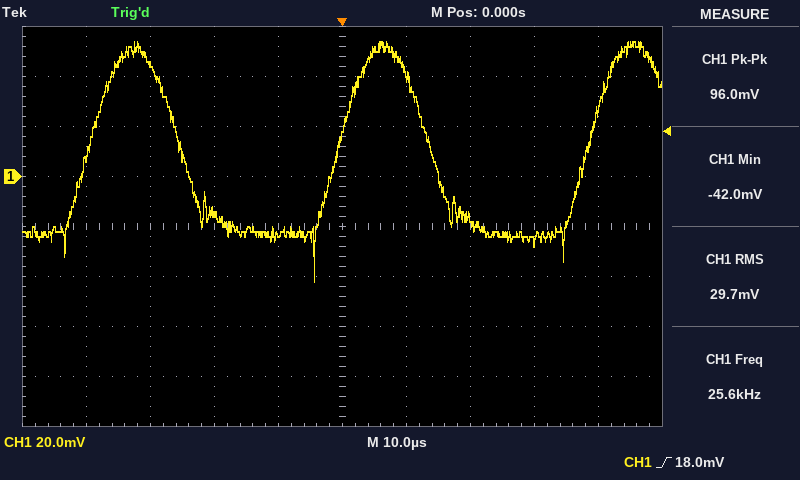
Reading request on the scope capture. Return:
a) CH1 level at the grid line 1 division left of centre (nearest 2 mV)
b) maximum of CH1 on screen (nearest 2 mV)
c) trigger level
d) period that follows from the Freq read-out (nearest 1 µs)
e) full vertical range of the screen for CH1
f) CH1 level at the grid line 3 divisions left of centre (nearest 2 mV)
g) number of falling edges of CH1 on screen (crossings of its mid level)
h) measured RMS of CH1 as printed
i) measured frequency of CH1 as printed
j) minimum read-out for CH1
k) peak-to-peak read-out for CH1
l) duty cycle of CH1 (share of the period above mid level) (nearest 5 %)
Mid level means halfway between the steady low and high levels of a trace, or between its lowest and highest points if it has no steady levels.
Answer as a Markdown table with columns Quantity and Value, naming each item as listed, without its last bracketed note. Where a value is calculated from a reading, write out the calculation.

| Quantity | Value |
|---|---|
| CH1 level at the grid line 1 division left of centre | -24 mV |
| maximum of CH1 on screen | 54 mV |
| trigger level | 18.0 mV |
| period that follows from the Freq read-out | 1 / 25.6 kHz ≈ 39 µs |
| full vertical range of the screen for CH1 | 160 mV |
| CH1 level at the grid line 3 divisions left of centre | 44 mV |
| number of falling edges of CH1 on screen | 2 |
| measured RMS of CH1 as printed | 29.7 mV |
| measured frequency of CH1 as printed | 25.6 kHz |
| minimum read-out for CH1 | -42.0 mV |
| peak-to-peak read-out for CH1 | 96.0 mV |
| duty cycle of CH1 (share of the period above mid level) | 40 % |
